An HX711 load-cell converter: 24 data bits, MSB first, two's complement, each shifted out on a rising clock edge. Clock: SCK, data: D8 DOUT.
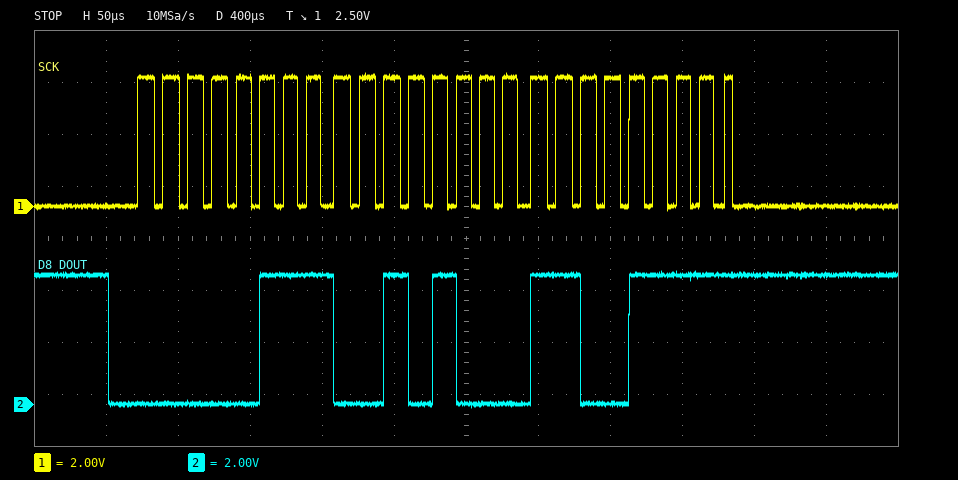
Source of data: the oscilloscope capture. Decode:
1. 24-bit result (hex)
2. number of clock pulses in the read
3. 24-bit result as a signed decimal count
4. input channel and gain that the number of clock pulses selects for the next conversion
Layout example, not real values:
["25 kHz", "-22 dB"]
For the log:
["0x0728CF", "25", "469199", "channel A, gain 128"]
